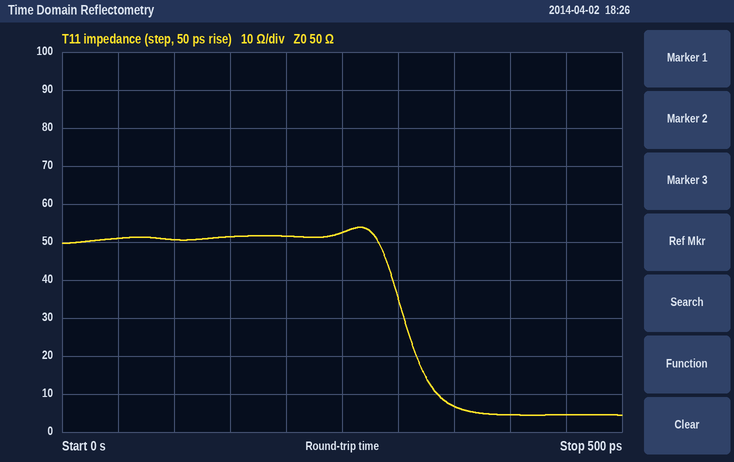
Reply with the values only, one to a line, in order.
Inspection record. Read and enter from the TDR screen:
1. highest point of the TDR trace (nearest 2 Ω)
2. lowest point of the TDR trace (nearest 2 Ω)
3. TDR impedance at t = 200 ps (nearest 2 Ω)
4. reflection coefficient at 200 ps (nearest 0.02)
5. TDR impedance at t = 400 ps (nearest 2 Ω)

54 Ω
4 Ω
52 Ω
+0.02
4 Ω
